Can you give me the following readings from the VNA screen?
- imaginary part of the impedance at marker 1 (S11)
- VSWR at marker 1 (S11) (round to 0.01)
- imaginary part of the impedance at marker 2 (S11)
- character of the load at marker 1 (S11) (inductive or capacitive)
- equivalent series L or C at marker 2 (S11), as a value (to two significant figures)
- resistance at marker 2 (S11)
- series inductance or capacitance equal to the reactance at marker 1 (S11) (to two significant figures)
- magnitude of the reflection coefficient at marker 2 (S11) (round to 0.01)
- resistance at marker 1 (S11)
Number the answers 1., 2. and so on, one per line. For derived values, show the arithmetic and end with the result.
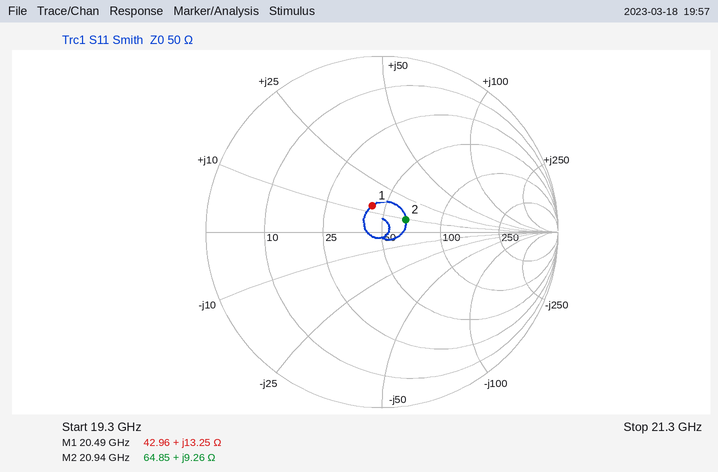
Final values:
1. +13.25 Ω
2. 1.38
3. +9.26 Ω
4. inductive
5. L = 9.26 Ω/(2π × 20.94 GHz) ≈ 70 pH
6. 64.85 Ω
7. L = 13.25 Ω/(2π × 20.49 GHz) ≈ 103 pH, so 100 pH to two significant figures
8. 0.15
9. 42.96 Ω
